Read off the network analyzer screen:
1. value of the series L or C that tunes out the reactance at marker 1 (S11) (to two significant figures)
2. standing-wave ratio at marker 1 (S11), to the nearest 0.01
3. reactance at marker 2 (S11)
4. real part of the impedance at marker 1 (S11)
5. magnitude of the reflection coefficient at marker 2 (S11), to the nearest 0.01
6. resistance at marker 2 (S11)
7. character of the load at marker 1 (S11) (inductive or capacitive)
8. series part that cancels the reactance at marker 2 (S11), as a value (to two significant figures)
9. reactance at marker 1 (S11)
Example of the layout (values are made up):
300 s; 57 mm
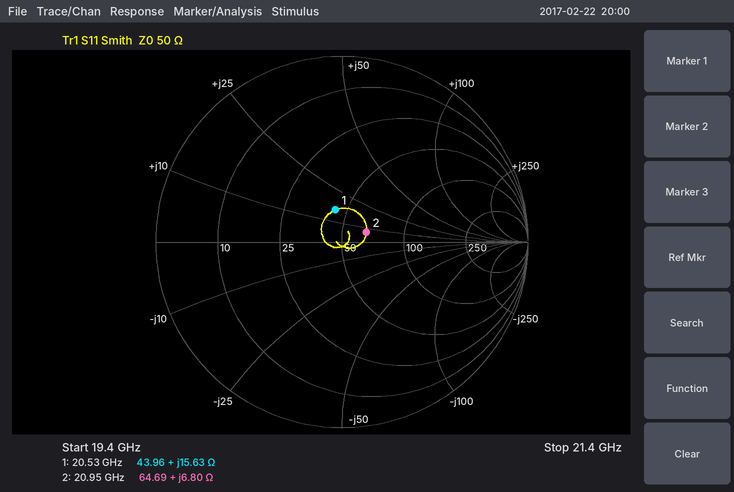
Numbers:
500 fF; 1.43; +6.80 Ω; 43.96 Ω; 0.14; 64.69 Ω; inductive; 1.1 pF; +15.63 Ω
